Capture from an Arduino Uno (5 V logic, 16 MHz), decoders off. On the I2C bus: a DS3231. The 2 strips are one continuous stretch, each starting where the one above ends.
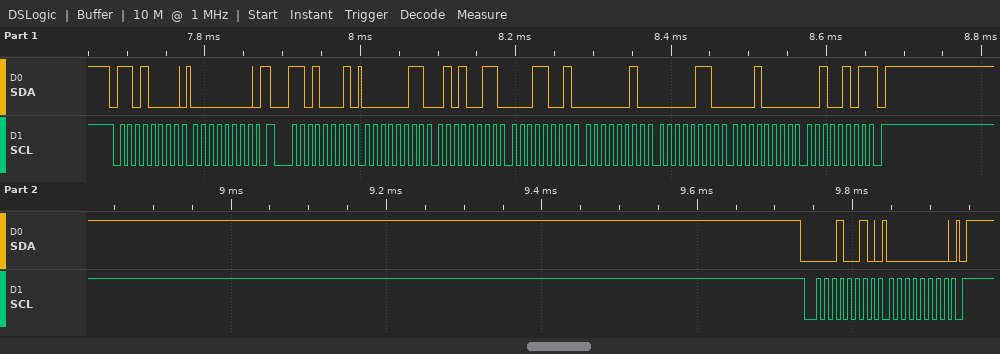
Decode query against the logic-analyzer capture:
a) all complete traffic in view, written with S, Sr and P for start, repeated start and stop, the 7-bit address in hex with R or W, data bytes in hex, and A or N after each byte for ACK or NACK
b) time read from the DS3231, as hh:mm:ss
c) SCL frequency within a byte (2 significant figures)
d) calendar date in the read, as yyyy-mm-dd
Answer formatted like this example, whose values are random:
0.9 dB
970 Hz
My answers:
S 68W A 00 A Sr 68R A 03 A 53 A 19 A 02 A 06 A 10 A 25 N P S 09W A 00 A P
19:53:03
100 kHz
2025-10-06
